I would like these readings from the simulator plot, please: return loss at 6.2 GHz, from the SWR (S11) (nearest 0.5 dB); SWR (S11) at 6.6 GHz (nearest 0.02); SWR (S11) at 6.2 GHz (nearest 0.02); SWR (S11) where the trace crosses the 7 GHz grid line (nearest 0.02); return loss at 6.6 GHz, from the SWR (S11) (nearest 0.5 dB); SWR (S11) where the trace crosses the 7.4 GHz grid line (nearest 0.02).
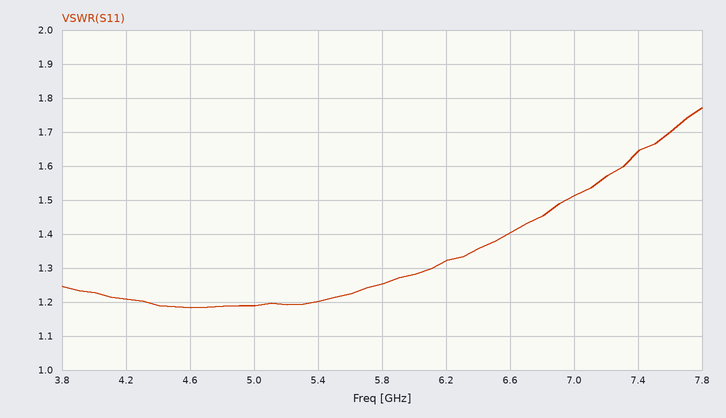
17.0 dB
1.40
1.32
1.52
15.5 dB
1.64
